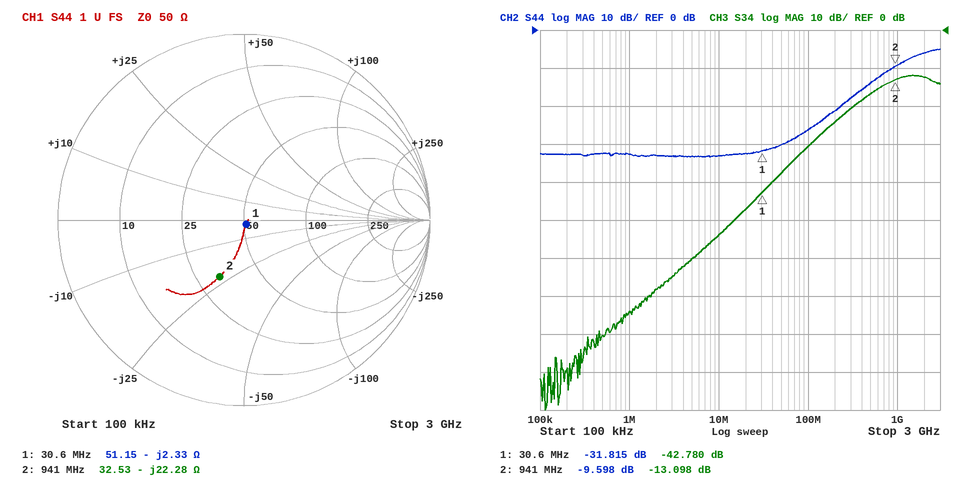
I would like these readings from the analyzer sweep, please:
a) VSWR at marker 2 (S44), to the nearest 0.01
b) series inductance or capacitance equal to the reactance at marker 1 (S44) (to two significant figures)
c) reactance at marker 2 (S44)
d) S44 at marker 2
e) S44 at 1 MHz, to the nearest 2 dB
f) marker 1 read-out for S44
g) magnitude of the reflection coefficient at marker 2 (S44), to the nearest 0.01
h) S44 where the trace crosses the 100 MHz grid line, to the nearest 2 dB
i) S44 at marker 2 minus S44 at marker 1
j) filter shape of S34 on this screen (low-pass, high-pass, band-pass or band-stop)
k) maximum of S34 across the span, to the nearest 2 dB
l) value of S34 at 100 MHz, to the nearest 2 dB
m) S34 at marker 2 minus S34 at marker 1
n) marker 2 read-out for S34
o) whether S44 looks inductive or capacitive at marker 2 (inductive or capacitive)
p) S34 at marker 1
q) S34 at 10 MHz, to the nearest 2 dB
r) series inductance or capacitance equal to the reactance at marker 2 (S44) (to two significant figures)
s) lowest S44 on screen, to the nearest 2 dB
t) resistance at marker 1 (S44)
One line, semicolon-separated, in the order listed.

1.99; 2.2 nF; -22.28 Ω; -9.598 dB; -32 dB; -31.815 dB; 0.33; -26 dB; 22.217 dB; high-pass; -12 dB; -30 dB; 29.682 dB; -13.098 dB; capacitive; -42.780 dB; -54 dB; 7.6 pF; -34 dB; 51.15 Ω
